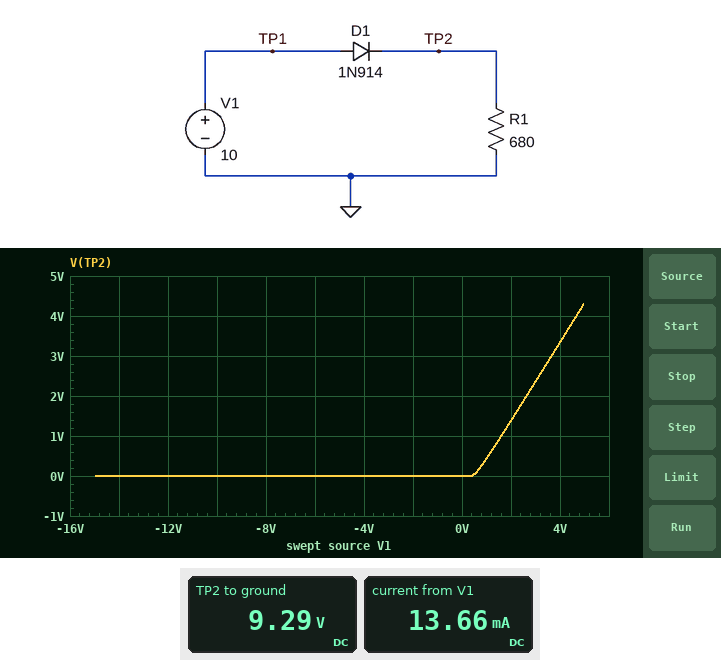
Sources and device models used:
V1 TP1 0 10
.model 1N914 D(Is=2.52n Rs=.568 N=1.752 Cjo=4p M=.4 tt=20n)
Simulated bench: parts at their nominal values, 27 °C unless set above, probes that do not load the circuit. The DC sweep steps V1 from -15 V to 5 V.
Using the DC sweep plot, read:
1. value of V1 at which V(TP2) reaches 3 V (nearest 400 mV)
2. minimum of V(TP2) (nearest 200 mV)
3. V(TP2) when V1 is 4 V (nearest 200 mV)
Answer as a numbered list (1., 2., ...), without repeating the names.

1. 3.6 V
2. 0 V
3. 3.4 V
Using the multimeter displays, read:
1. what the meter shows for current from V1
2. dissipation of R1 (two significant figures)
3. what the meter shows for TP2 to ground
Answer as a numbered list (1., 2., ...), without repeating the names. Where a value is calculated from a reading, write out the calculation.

1. 13.66 mA
2. (9.29 V)^2 / 680 Ω = 130 mW
3. 9.29 V
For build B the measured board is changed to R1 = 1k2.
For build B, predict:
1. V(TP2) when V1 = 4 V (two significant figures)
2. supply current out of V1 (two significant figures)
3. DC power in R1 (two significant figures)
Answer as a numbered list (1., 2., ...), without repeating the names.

1. 3.4 V
2. 7.8 mA
3. 72 mW
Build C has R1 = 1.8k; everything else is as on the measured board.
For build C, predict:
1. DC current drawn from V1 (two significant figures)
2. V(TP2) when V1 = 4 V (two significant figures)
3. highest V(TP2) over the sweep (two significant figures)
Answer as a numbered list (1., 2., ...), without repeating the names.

1. 5.2 mA
2. 3.4 V
3. 4.4 V
